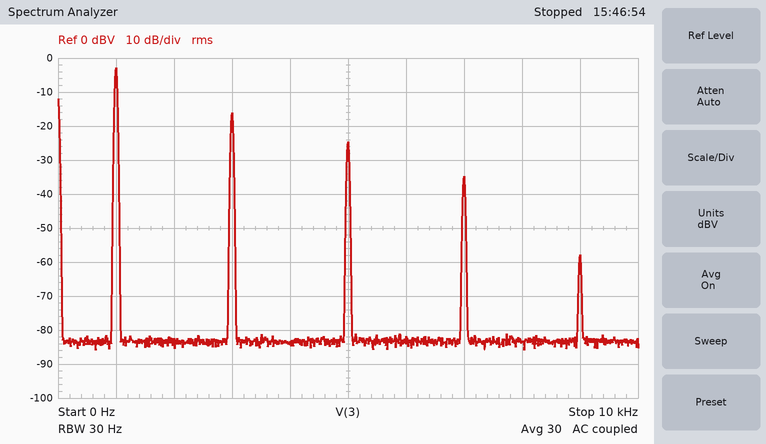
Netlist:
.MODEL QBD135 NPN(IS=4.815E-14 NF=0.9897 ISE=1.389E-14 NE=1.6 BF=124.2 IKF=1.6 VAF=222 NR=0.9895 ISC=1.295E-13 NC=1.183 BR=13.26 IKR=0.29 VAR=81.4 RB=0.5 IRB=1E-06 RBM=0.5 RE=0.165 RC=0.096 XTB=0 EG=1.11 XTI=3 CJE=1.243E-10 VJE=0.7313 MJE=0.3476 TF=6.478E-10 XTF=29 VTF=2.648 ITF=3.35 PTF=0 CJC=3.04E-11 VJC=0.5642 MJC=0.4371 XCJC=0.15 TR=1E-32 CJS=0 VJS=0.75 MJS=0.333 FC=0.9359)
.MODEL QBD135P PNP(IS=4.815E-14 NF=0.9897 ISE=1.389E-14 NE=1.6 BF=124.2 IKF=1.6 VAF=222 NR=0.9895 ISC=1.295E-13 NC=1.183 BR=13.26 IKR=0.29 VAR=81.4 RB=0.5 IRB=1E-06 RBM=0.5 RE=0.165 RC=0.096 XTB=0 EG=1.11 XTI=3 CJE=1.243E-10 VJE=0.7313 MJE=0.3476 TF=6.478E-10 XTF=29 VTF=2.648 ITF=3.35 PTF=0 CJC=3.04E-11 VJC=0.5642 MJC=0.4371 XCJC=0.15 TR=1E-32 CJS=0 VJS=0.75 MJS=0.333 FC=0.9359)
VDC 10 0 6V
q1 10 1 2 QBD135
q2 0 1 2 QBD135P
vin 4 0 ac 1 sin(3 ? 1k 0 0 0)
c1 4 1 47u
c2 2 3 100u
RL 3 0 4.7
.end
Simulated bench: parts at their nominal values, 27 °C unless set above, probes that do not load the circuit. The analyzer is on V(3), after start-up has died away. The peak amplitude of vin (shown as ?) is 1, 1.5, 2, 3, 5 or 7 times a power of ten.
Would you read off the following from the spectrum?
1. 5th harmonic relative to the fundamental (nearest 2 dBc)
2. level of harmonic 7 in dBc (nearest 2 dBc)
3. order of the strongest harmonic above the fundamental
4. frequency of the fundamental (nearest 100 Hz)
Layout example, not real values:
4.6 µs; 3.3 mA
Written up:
-22 dBc; -32 dBc; 3; 1.0 kHz
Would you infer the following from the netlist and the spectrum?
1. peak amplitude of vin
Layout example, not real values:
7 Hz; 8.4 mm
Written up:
2 V
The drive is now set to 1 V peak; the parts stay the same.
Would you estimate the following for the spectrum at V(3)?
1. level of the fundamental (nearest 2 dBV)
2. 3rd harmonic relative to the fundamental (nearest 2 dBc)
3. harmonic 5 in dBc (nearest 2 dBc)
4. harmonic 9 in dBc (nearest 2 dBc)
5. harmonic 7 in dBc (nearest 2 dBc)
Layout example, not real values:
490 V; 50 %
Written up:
-18 dBV; -6 dBc; -24 dBc; -44 dBc; -24 dBc
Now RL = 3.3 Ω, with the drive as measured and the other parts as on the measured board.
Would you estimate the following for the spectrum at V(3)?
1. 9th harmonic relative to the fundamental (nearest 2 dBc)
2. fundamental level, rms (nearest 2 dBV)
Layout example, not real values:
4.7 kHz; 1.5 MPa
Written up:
-50 dBc; -4 dBV
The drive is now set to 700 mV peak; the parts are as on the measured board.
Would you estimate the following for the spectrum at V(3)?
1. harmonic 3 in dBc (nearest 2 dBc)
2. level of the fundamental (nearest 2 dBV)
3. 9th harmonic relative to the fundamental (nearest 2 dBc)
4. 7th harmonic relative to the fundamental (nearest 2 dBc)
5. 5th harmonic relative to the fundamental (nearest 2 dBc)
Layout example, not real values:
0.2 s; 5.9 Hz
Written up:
-2 dBc; -40 dBV; -30 dBc; -14 dBc; -6 dBc
